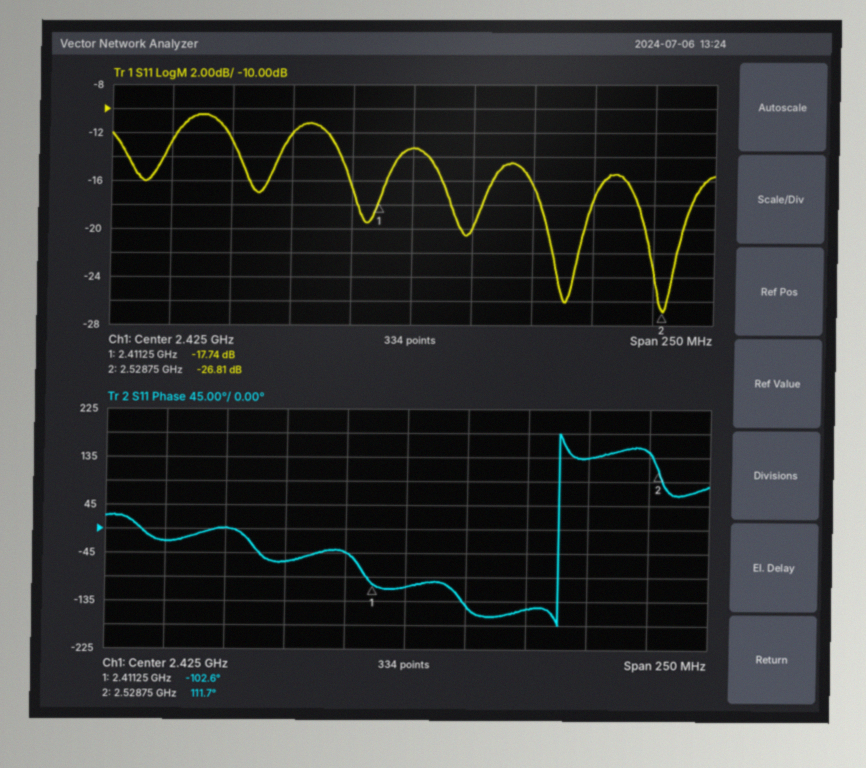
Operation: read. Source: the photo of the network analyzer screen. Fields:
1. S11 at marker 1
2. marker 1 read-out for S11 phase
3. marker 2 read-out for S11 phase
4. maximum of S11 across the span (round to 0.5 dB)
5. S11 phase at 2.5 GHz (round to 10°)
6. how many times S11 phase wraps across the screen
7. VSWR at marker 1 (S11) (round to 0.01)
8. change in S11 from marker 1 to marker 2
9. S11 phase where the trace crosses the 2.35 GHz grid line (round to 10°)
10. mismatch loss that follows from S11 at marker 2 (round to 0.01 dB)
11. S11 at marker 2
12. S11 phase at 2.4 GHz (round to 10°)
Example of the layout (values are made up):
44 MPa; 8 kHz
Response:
-17.74 dB; -102.6°; 111.7°; -10.5 dB; 130°; 1; 1.30; -9.07 dB; 0°; 0.01 dB; -26.81 dB; -40°
